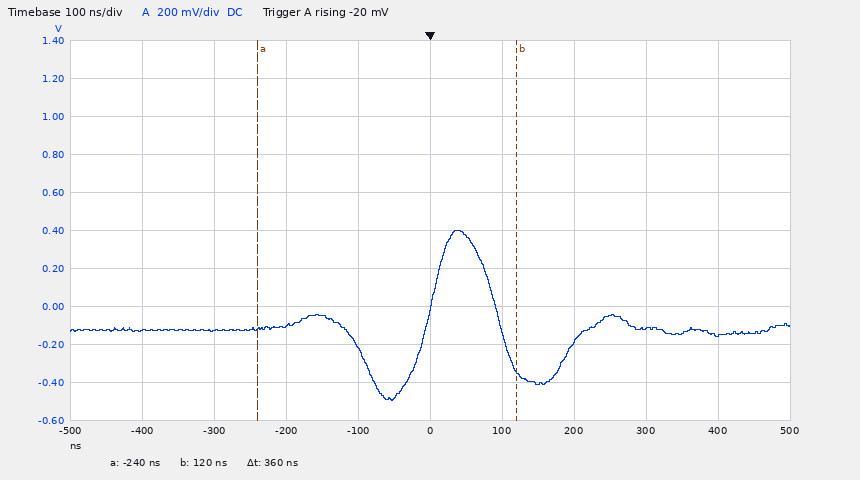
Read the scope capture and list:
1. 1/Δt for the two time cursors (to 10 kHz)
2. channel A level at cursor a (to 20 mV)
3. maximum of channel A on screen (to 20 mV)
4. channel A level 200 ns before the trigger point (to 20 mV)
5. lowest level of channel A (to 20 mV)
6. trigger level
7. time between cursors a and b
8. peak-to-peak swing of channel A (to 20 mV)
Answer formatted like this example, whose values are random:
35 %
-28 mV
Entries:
2.78 MHz
-120 mV
400 mV
-100 mV
-500 mV
-20 mV
360 ns
900 mV
